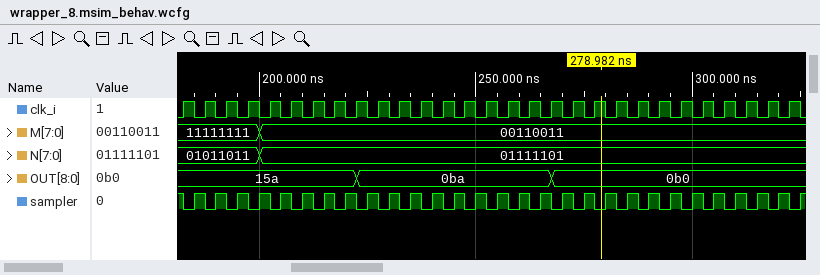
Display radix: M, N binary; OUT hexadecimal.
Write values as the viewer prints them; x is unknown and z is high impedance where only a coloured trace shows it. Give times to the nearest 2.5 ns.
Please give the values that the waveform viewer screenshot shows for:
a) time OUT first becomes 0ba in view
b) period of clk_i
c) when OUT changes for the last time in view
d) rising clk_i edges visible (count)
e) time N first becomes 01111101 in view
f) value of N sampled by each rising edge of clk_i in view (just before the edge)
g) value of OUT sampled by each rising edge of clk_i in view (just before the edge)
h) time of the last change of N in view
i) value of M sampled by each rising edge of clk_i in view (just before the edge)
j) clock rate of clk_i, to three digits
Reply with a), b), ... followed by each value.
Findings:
a) 222.5 ns
b) 5 ns
c) 267.5 ns
d) 29
e) 200 ns
f) 01011011, 01011011, 01011011, 01011011, 01111101, 01111101, 01111101, 01111101, 01111101, 01111101, 01111101, 01111101, 01111101, 01111101, 01111101, 01111101, 01111101, 01111101, 01111101, 01111101, 01111101, 01111101, 01111101, 01111101, 01111101, 01111101, 01111101, 01111101, 01111101
g) 15a, 15a, 15a, 15a, 15a, 15a, 15a, 15a, 15a, 0ba, 0ba, 0ba, 0ba, 0ba, 0ba, 0ba, 0ba, 0ba, 0b0, 0b0, 0b0, 0b0, 0b0, 0b0, 0b0, 0b0, 0b0, 0b0, 0b0
h) 200 ns
i) 11111111, 11111111, 11111111, 11111111, 00110011, 00110011, 00110011, 00110011, 00110011, 00110011, 00110011, 00110011, 00110011, 00110011, 00110011, 00110011, 00110011, 00110011, 00110011, 00110011, 00110011, 00110011, 00110011, 00110011, 00110011, 00110011, 00110011, 00110011, 00110011
j) 200 MHz
